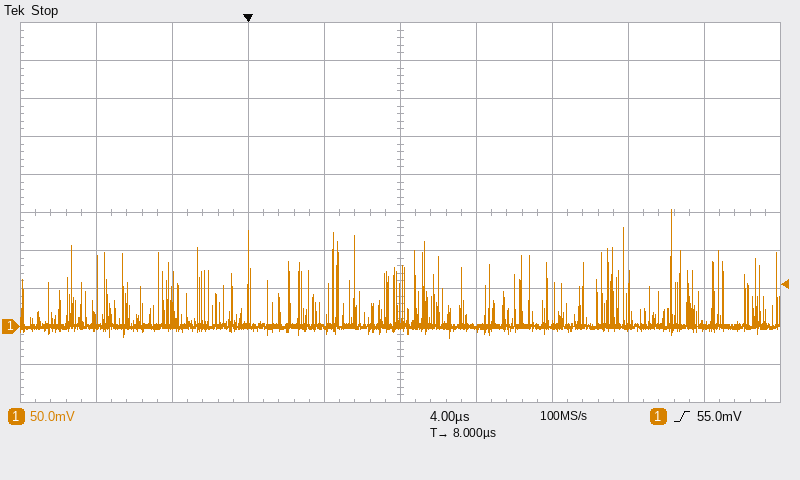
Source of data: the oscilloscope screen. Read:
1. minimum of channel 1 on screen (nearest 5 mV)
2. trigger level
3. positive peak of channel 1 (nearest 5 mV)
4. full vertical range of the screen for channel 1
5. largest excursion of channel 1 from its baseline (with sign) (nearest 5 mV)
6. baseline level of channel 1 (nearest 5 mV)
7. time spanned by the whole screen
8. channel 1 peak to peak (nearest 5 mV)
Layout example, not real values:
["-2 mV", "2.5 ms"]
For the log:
["-15 mV", "55.0 mV", "155 mV", "500 mV", "+155 mV", "0 mV", "40 µs", "170 mV"]
